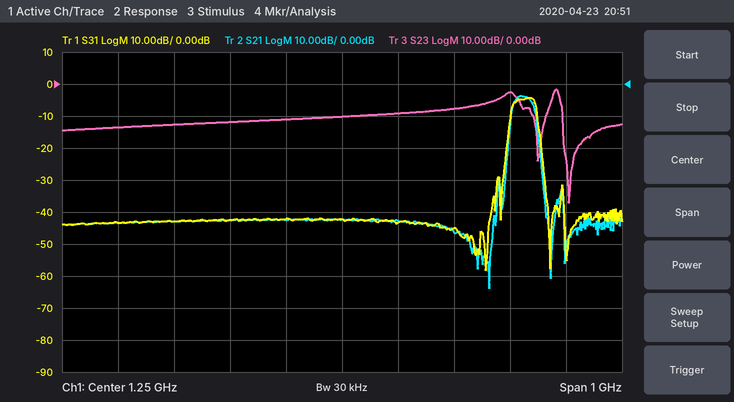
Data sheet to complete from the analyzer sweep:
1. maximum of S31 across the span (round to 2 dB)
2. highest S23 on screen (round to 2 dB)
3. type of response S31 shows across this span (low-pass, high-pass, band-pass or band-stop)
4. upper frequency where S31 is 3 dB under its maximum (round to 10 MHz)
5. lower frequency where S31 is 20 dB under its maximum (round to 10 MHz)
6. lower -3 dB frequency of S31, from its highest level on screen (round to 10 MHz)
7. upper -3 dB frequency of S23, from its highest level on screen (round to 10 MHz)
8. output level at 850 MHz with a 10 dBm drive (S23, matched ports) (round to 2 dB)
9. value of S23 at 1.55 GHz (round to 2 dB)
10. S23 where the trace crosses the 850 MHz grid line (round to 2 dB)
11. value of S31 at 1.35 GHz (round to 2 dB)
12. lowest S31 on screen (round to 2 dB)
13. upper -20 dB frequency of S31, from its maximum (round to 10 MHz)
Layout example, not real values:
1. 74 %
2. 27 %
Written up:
1. -4 dB
2. -2 dB
3. band-pass
4. 1.60 GHz
5. 1.54 GHz
6. 1.55 GHz
7. 1.64 GHz
8. -4 dBm
9. -2 dB
10. -14 dB
11. -44 dB
12. -58 dB
13. 1.61 GHz
